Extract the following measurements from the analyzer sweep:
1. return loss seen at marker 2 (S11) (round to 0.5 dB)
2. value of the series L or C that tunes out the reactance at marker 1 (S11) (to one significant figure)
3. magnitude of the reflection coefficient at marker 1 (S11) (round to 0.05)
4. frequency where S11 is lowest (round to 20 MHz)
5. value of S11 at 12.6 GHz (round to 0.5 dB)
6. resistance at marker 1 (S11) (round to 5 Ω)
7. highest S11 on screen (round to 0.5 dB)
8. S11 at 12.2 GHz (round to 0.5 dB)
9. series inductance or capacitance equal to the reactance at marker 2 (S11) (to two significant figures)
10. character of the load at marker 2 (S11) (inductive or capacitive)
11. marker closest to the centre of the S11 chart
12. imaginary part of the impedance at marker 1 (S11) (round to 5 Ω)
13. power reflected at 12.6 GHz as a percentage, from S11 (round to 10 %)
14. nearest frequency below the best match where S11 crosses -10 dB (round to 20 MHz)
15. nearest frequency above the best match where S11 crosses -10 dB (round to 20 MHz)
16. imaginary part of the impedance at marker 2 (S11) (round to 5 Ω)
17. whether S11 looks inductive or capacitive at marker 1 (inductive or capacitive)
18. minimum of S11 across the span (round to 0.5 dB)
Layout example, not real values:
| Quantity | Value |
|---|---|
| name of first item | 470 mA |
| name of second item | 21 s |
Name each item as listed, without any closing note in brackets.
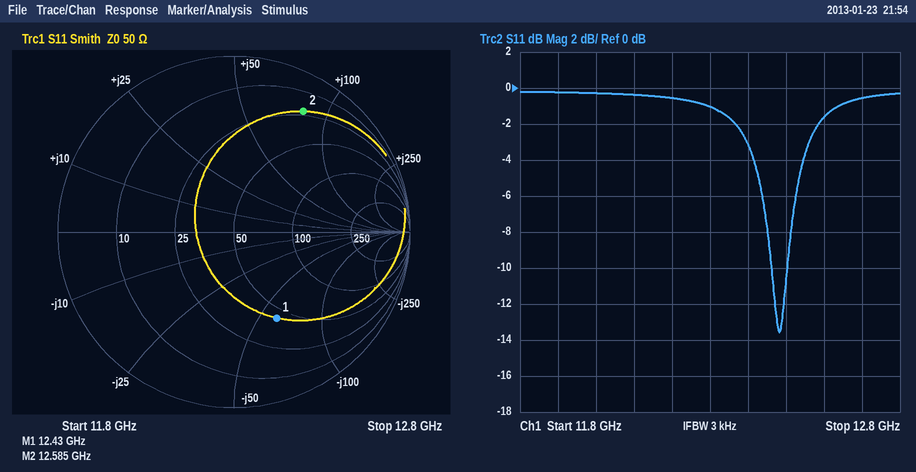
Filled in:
| Quantity | Value |
|---|---|
| return loss seen at marker 2 (S11) | 2.0 dB |
| value of the series L or C that tunes out the reactance at marker 1 (S11) | 800 pH |
| magnitude of the reflection coefficient at marker 1 (S11) | 0.55 |
| frequency where S11 is lowest | 12.48 GHz |
| value of S11 at 12.6 GHz | -1.5 dB |
| resistance at marker 1 (S11) | 45 Ω |
| highest S11 on screen | 0.0 dB |
| S11 at 12.2 GHz | -0.5 dB |
| series inductance or capacitance equal to the reactance at marker 2 (S11) | 1.0 nH |
| character of the load at marker 2 (S11) | inductive |
| marker closest to the centre of the S11 chart | marker 1 |
| imaginary part of the impedance at marker 1 (S11) | -60 Ω |
| power reflected at 12.6 GHz as a percentage, from S11 | 70 % |
| nearest frequency below the best match where S11 crosses -10 dB | 12.46 GHz |
| nearest frequency above the best match where S11 crosses -10 dB | 12.50 GHz |
| imaginary part of the impedance at marker 2 (S11) | +80 Ω |
| whether S11 looks inductive or capacitive at marker 1 | capacitive |
| minimum of S11 across the span | -13.5 dB |
